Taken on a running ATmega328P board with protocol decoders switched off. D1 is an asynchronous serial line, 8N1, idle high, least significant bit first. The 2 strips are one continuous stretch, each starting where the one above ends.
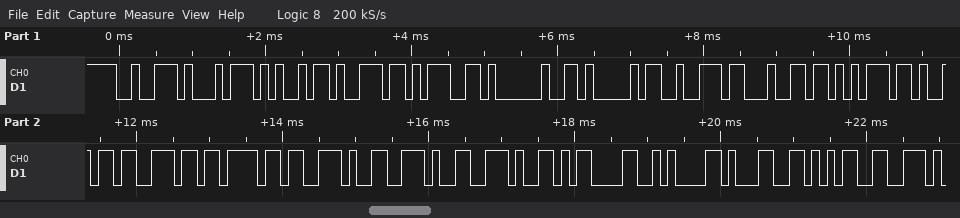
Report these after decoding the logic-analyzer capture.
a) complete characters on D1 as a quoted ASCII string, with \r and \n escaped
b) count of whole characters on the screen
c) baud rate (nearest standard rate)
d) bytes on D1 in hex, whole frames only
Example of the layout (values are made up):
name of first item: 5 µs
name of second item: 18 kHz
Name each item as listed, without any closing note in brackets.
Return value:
complete characters on D1 as a quoted ASCII string, with \r and \n escaped: "rting Arduino...\r\n15"
count of whole characters on the screen: 20
baud rate: 9600 baud
bytes on D1 in hex, whole frames only: 0x72 0x74 0x69 0x6E 0x67 0x20 0x41 0x72 0x64 0x75 0x69 0x6E 0x6F 0x2E 0x2E 0x2E 0x0D 0x0A 0x31 0x35
